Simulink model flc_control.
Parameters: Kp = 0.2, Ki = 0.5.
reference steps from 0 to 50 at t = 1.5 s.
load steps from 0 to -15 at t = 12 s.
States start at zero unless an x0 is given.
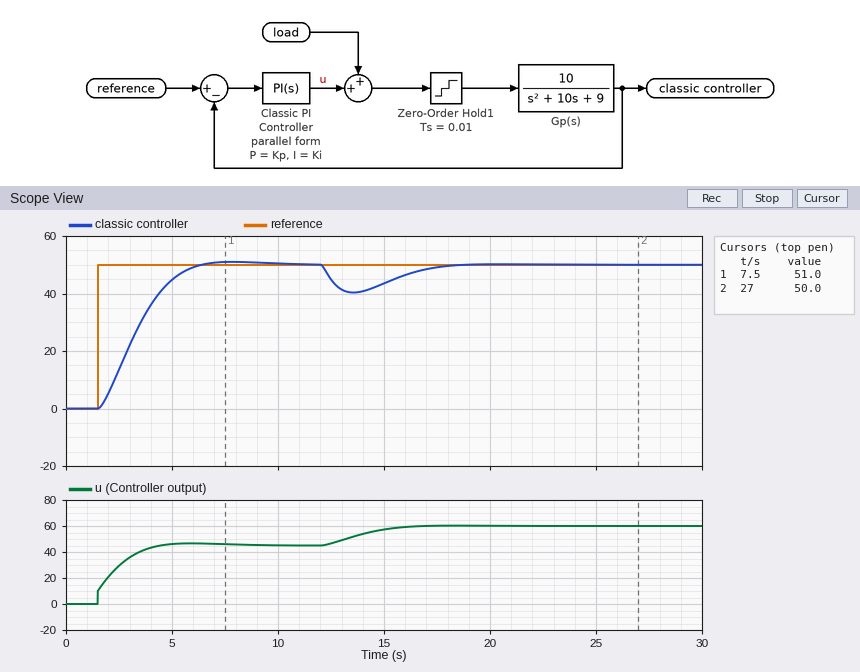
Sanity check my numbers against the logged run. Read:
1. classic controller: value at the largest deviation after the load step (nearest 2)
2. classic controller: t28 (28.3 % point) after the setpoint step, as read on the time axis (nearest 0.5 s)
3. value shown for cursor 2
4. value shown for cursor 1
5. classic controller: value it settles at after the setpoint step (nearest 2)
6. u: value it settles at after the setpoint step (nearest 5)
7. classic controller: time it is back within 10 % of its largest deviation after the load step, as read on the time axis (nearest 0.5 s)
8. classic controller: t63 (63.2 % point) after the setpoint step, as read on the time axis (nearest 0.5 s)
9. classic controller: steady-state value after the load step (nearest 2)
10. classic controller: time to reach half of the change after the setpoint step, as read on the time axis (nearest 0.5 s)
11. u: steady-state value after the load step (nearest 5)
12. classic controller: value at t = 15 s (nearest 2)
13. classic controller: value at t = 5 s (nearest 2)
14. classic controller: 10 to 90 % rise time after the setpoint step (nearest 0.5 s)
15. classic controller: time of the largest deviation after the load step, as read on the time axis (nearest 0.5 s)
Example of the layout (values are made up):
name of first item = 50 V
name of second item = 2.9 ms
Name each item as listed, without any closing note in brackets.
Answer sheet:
classic controller: value at the largest deviation after the load step = 40
classic controller: t28 (28.3 % point) after the setpoint step, as read on the time axis = 2.5 s
value shown for cursor 2 = 50.0
value shown for cursor 1 = 51.0
classic controller: value it settles at after the setpoint step = 50
u: value it settles at after the setpoint step = 45
classic controller: time it is back within 10 % of its largest deviation after the load step, as read on the time axis = 17.5 s
classic controller: t63 (63.2 % point) after the setpoint step, as read on the time axis = 3.5 s
classic controller: steady-state value after the load step = 50
classic controller: time to reach half of the change after the setpoint step, as read on the time axis = 3.0 s
u: steady-state value after the load step = 60
classic controller: value at t = 15 s = 44
classic controller: value at t = 5 s = 44
classic controller: 10 to 90 % rise time after the setpoint step = 3.0 s
classic controller: time of the largest deviation after the load step, as read on the time axis = 13.5 s
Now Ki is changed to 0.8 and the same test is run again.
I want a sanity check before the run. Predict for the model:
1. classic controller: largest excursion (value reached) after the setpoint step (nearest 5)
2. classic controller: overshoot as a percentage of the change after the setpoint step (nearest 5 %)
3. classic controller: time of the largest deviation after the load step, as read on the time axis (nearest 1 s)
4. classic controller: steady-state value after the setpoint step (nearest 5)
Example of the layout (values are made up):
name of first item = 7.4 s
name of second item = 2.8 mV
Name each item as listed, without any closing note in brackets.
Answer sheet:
classic controller: largest excursion (value reached) after the setpoint step = 55
classic controller: overshoot as a percentage of the change after the setpoint step = 10 %
classic controller: time of the largest deviation after the load step, as read on the time axis = 13 s
classic controller: steady-state value after the setpoint step = 50
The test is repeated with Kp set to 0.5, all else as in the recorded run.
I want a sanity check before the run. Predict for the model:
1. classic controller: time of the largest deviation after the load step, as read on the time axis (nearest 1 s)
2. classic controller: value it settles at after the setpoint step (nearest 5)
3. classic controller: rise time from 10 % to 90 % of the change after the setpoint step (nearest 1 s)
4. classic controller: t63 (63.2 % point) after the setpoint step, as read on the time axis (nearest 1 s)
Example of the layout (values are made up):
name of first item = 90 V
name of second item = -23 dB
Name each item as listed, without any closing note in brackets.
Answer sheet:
classic controller: time of the largest deviation after the load step, as read on the time axis = 13 s
classic controller: value it settles at after the setpoint step = 50
classic controller: rise time from 10 % to 90 % of the change after the setpoint step = 4 s
classic controller: t63 (63.2 % point) after the setpoint step, as read on the time axis = 3 s
